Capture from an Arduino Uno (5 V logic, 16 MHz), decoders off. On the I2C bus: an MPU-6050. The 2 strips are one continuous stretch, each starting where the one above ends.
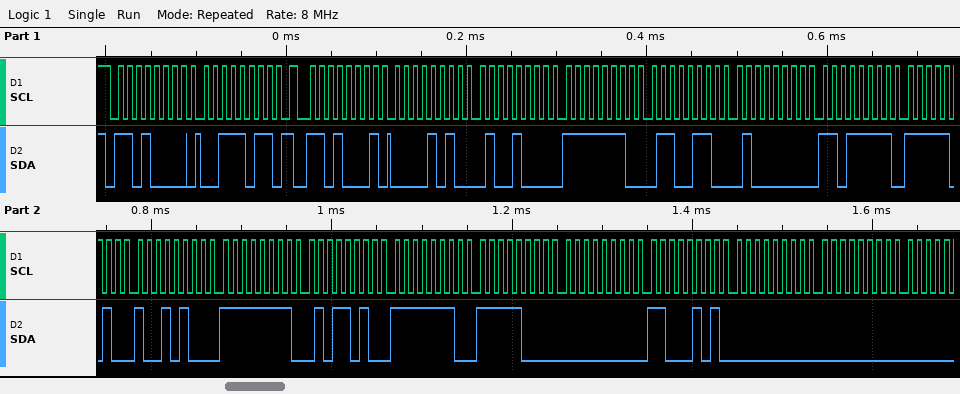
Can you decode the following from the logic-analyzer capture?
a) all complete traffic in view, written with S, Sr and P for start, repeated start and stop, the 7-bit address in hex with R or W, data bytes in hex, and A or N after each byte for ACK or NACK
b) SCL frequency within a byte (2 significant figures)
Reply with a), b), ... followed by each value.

a) S 68W A 3B A Sr 68R A 0A A 48 A FE A 66 A 40 A DF A FA A 94 A FF A 5A A FE A F8 A 00 A C5 A 00 A 00 A
b) 100 kHz
